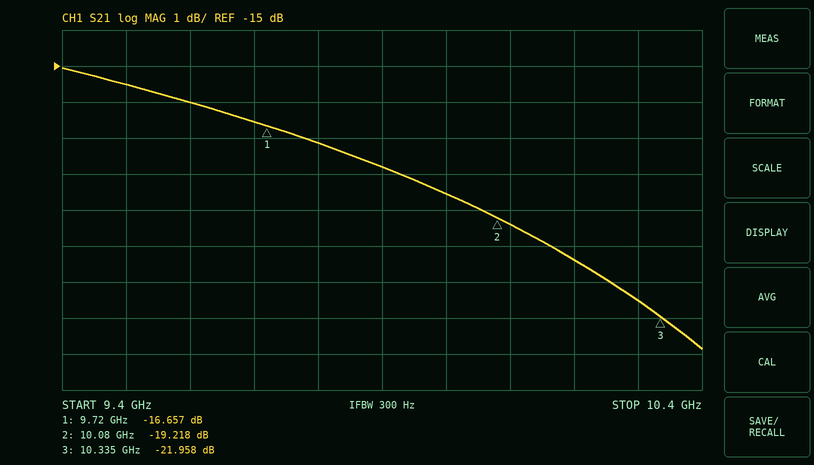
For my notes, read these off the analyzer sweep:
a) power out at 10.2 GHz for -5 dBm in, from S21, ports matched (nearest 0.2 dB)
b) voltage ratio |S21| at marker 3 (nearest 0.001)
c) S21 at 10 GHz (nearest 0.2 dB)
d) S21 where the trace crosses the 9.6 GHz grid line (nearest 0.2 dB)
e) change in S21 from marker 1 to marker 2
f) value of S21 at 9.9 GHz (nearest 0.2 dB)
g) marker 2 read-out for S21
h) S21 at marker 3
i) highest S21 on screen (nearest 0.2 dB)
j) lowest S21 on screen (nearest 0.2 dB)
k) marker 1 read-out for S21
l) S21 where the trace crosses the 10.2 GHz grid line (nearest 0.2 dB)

-25.4 dBm
0.080
-18.6 dB
-16.0 dB
-2.561 dB
-17.8 dB
-19.218 dB
-21.958 dB
-15.0 dB
-22.8 dB
-16.657 dB
-20.4 dB
